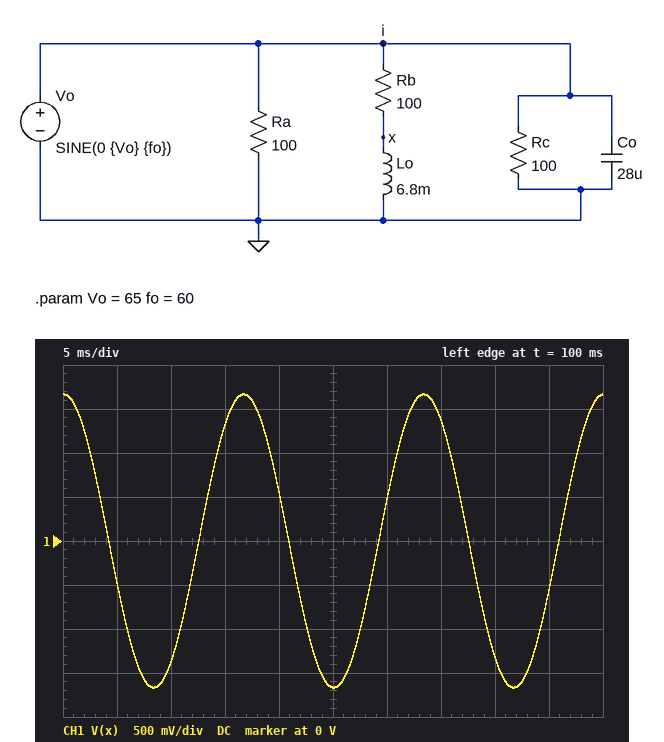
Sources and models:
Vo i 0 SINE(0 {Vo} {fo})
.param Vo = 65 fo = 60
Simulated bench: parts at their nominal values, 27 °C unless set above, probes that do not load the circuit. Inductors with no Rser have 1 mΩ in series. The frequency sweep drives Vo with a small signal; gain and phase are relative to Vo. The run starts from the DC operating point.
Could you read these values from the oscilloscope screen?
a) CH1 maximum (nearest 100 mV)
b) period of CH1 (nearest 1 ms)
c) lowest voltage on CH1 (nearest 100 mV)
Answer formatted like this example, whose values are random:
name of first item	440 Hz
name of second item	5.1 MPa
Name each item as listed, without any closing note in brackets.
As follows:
CH1 maximum	1.7 V
period of CH1	17 ms
lowest voltage on CH1	-1.7 V
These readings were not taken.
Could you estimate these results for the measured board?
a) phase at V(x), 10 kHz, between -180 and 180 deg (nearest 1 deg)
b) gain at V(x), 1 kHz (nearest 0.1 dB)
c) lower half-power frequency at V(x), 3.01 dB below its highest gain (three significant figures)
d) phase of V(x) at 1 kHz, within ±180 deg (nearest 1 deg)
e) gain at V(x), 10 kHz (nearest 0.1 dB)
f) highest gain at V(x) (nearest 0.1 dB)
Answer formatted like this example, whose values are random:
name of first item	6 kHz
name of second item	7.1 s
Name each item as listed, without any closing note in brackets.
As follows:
phase at V(x), 10 kHz, between -180 and 180 deg	13 deg
gain at V(x), 1 kHz	-8.1 dB
lower half-power frequency at V(x), 3.01 dB below its highest gain	2.34 kHz
phase of V(x) at 1 kHz, within ±180 deg	67 deg
gain at V(x), 10 kHz	-0.2 dB
highest gain at V(x)	0 dB
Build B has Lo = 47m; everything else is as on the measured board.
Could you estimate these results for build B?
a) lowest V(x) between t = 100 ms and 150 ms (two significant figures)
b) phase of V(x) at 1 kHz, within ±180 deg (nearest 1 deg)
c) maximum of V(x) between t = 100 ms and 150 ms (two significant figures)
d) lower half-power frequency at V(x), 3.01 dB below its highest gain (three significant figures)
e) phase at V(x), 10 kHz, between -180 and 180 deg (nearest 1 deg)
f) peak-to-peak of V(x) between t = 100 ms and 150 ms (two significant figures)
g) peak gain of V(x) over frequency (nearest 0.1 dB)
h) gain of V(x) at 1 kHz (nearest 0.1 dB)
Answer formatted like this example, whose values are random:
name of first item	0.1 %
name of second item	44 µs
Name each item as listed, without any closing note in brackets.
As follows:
lowest V(x) between t = 100 ms and 150 ms	-11 V
phase of V(x) at 1 kHz, within ±180 deg	19 deg
maximum of V(x) between t = 100 ms and 150 ms	11 V
lower half-power frequency at V(x), 3.01 dB below its highest gain	339 Hz
phase at V(x), 10 kHz, between -180 and 180 deg	2 deg
peak-to-peak of V(x) between t = 100 ms and 150 ms	23 V
peak gain of V(x) over frequency	0 dB
gain of V(x) at 1 kHz	-0.5 dB
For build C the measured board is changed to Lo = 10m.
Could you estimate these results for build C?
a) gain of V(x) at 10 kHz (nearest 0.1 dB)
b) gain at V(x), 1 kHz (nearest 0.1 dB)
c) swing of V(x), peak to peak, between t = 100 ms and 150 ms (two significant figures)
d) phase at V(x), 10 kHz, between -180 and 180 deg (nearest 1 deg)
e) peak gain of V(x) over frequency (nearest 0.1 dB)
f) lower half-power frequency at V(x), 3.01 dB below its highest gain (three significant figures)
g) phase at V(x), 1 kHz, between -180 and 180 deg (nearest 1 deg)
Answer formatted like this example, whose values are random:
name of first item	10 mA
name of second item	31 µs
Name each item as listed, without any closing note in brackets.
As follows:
gain of V(x) at 10 kHz	-0.1 dB
gain at V(x), 1 kHz	-5.5 dB
swing of V(x), peak to peak, between t = 100 ms and 150 ms	4.9 V
phase at V(x), 10 kHz, between -180 and 180 deg	9 deg
peak gain of V(x) over frequency	0 dB
lower half-power frequency at V(x), 3.01 dB below its highest gain	1.59 kHz
phase at V(x), 1 kHz, between -180 and 180 deg	58 deg
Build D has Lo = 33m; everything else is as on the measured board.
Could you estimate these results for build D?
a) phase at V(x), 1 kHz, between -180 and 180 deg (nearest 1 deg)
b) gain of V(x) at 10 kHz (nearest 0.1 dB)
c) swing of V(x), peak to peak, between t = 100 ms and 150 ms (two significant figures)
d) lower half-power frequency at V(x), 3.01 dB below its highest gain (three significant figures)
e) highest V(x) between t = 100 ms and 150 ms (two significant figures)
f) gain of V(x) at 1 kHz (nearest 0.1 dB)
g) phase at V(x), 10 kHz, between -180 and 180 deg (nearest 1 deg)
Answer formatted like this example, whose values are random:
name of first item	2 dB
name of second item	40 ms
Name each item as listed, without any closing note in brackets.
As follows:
phase at V(x), 1 kHz, between -180 and 180 deg	26 deg
gain of V(x) at 10 kHz	0 dB
swing of V(x), peak to peak, between t = 100 ms and 150 ms	16 V
lower half-power frequency at V(x), 3.01 dB below its highest gain	482 Hz
highest V(x) between t = 100 ms and 150 ms	8.0 V
gain of V(x) at 1 kHz	-0.9 dB
phase at V(x), 10 kHz, between -180 and 180 deg	3 deg
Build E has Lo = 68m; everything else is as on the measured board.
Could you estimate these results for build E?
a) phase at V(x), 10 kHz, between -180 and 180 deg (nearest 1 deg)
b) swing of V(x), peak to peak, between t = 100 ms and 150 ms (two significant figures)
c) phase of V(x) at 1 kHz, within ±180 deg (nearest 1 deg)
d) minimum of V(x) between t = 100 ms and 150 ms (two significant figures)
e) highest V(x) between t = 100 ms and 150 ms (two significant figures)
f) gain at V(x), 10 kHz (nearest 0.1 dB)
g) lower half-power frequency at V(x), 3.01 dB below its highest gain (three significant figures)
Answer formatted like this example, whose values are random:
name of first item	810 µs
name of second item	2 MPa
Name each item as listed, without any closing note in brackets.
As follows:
phase at V(x), 10 kHz, between -180 and 180 deg	1 deg
swing of V(x), peak to peak, between t = 100 ms and 150 ms	32 V
phase of V(x) at 1 kHz, within ±180 deg	13 deg
minimum of V(x) between t = 100 ms and 150 ms	-16 V
highest V(x) between t = 100 ms and 150 ms	16 V
gain at V(x), 10 kHz	0 dB
lower half-power frequency at V(x), 3.01 dB below its highest gain	234 Hz
